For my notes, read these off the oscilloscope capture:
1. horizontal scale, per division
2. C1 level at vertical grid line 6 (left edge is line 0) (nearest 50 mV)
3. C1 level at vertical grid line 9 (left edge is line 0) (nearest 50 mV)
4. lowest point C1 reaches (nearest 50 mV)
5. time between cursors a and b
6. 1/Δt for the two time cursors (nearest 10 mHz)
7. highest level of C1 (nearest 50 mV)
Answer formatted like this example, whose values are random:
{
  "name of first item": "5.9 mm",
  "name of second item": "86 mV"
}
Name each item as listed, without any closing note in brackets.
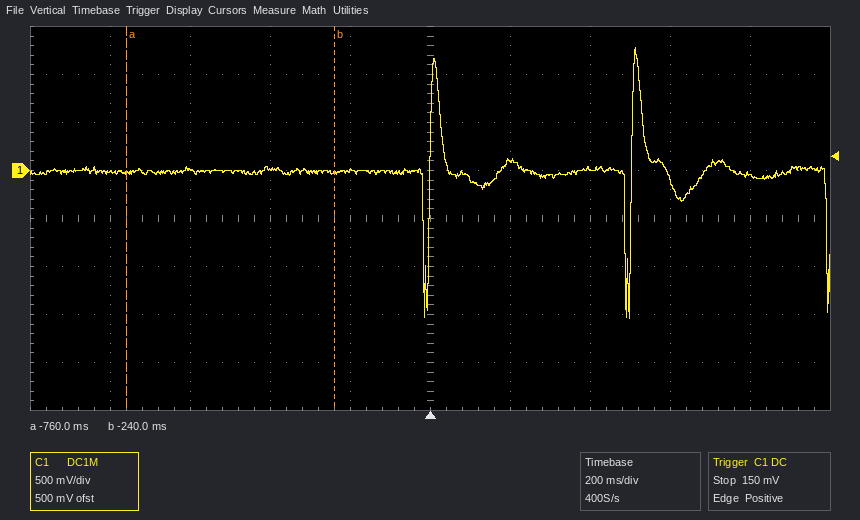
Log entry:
{
  "horizontal scale, per division": "200 ms",
  "C1 level at vertical grid line 6 (left edge is line 0)": "100 mV",
  "C1 level at vertical grid line 9 (left edge is line 0)": "-50 mV",
  "lowest point C1 reaches": "-1.55 V",
  "time between cursors a and b": "520 ms",
  "1/Δt for the two time cursors": "1.92 Hz",
  "highest level of C1": "1.30 V"
}
